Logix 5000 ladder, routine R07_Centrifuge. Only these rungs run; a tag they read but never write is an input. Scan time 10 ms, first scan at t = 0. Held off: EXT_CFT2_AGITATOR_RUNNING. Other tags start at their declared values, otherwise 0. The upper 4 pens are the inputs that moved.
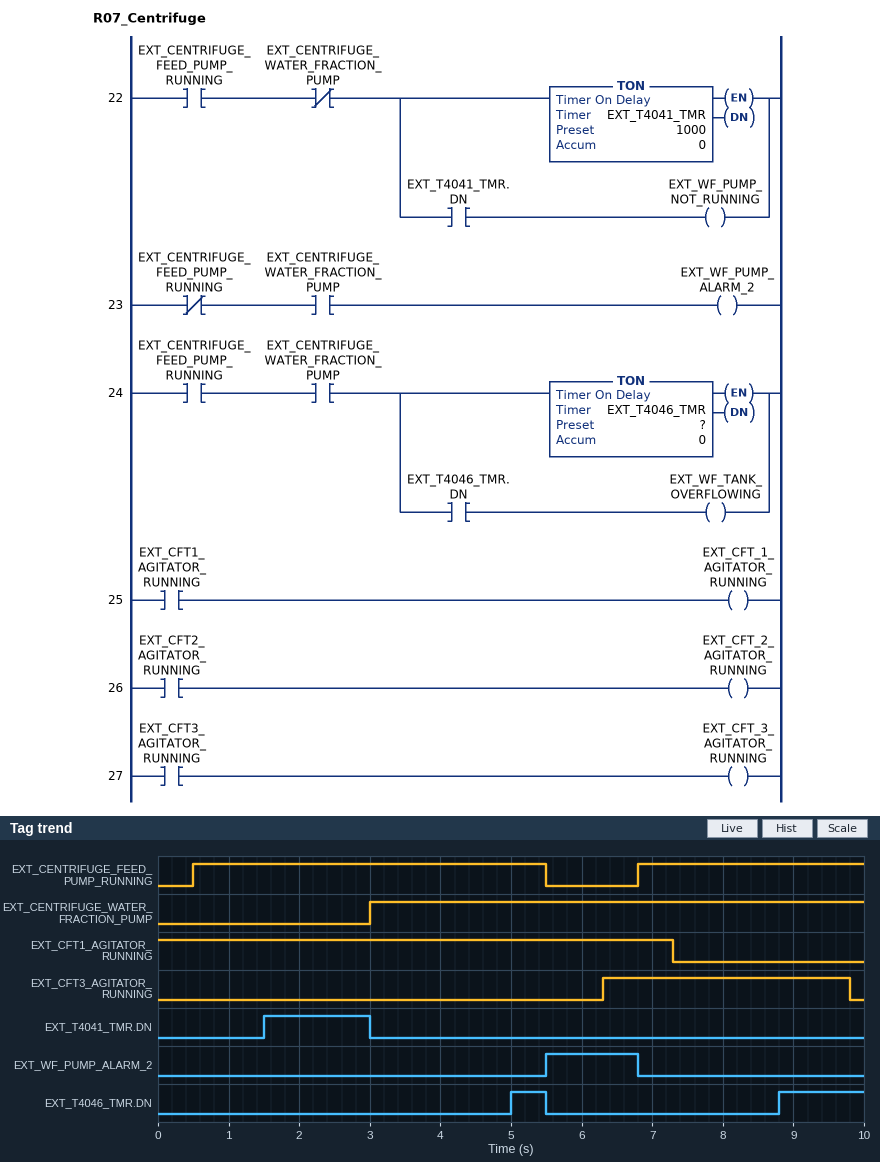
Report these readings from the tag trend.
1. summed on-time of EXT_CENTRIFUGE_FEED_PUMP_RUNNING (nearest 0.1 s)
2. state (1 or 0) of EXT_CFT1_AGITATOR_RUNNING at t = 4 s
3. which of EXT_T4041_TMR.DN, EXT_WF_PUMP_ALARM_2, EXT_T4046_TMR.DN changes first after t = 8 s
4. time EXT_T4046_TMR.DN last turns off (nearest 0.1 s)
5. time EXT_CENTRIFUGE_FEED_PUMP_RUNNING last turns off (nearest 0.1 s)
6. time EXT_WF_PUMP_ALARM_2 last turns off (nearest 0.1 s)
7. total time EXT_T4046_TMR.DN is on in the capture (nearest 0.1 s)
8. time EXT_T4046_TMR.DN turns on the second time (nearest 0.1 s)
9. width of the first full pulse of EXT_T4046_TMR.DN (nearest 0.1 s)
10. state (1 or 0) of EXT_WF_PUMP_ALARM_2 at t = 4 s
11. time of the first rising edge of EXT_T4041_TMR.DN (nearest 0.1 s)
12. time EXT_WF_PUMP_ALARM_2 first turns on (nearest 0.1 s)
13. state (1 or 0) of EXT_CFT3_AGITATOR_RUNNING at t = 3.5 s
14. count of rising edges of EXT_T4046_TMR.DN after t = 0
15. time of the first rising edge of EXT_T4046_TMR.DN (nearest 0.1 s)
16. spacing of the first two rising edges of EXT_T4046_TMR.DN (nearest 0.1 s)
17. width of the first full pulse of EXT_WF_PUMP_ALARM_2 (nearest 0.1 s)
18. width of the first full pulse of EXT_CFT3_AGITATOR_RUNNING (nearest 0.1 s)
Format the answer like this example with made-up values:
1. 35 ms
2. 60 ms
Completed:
1. 8.2 s
2. 1
3. EXT_T4046_TMR.DN
4. 5.5 s
5. 5.5 s
6. 6.8 s
7. 1.7 s
8. 8.8 s
9. 0.5 s
10. 0
11. 1.5 s
12. 5.5 s
13. 0
14. 2
15. 5.0 s
16. 3.8 s
17. 1.3 s
18. 3.5 s
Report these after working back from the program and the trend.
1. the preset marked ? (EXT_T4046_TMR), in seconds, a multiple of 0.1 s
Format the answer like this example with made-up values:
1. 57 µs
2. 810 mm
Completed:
1. 2.0 s
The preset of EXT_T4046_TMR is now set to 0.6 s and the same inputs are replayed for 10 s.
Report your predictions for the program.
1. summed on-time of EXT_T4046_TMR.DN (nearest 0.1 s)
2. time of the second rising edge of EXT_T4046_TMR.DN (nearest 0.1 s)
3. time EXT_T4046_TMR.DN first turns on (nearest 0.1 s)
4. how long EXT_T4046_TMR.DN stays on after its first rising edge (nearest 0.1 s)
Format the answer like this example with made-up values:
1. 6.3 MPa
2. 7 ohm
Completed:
1. 4.5 s
2. 7.4 s
3. 3.6 s
4. 1.9 s
